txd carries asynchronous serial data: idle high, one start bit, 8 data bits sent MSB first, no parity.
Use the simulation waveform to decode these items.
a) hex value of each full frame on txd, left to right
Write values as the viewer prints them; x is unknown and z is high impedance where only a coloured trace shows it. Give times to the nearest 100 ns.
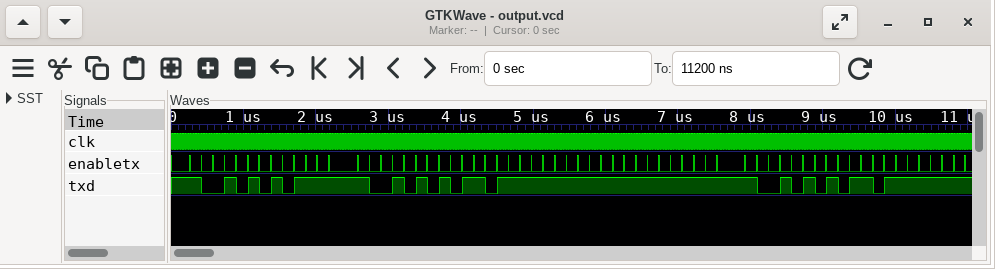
55, 55, FF, 55
